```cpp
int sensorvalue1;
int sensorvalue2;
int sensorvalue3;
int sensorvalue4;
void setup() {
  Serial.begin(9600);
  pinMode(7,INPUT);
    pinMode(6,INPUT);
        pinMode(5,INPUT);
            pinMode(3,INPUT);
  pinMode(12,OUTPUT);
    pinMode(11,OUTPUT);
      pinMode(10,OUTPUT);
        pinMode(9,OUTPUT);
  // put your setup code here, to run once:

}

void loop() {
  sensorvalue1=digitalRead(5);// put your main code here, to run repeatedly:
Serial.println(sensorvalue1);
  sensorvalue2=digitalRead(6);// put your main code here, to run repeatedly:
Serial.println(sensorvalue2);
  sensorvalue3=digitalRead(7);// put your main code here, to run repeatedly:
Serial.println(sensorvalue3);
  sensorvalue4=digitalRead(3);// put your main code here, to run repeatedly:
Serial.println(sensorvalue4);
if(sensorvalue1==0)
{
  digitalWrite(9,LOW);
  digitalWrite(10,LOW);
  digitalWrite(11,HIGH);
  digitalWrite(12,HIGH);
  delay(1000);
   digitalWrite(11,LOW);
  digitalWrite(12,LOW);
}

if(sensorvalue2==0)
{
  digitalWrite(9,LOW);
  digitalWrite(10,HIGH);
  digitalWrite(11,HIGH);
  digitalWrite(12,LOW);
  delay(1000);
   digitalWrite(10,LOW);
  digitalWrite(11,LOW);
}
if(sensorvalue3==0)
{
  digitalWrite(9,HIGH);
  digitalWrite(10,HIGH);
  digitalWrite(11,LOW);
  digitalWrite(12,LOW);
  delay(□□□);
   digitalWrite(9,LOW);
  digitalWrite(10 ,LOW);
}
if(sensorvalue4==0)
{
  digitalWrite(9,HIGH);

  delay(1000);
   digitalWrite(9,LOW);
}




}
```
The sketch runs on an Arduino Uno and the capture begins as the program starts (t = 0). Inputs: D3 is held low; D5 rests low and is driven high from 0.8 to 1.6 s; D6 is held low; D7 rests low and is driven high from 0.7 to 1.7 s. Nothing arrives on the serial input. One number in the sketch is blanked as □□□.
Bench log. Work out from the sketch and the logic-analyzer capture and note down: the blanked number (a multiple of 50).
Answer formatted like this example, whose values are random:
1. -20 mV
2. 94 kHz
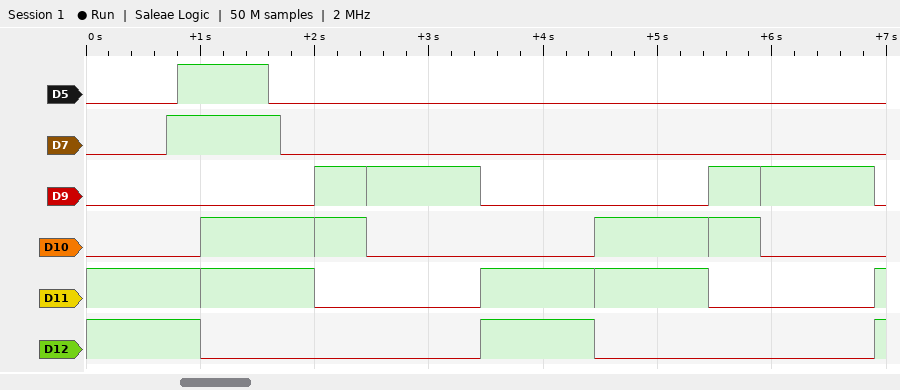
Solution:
1. 450
